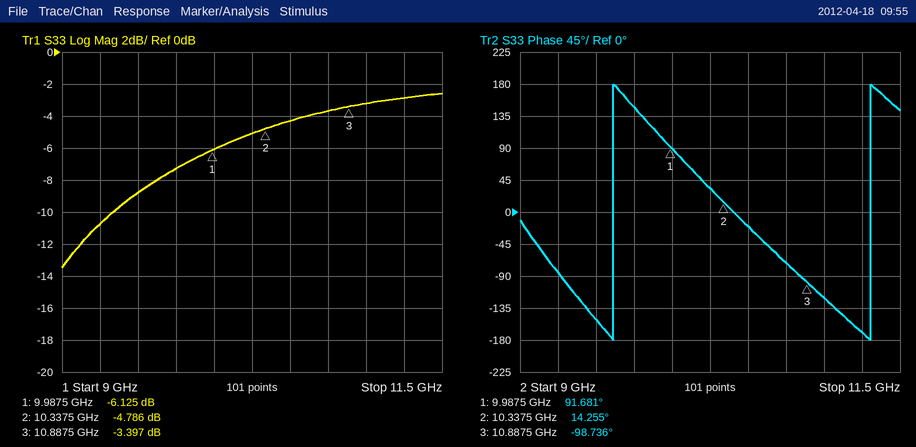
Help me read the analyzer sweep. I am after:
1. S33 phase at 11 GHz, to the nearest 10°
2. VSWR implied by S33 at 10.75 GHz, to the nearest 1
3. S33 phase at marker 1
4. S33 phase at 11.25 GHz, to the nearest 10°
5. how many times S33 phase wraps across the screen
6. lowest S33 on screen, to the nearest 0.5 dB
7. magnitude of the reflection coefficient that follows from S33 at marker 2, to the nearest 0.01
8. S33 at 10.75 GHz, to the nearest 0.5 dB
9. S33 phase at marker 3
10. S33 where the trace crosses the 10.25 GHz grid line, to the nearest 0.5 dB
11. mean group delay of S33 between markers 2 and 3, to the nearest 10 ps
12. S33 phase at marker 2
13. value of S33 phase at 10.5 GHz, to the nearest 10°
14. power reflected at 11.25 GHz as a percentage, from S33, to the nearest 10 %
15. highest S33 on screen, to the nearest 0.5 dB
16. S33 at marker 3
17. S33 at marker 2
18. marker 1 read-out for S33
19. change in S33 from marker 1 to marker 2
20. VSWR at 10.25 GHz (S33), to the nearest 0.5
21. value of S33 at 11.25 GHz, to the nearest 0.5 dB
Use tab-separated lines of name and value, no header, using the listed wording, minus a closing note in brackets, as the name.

S33 phase at 11 GHz, to the nearest 10°	-120°
VSWR implied by S33 at 10.75 GHz, to the nearest 1	5
S33 phase at marker 1	91.681°
S33 phase at 11.25 GHz, to the nearest 10°	-170°
how many times S33 phase wraps across the screen	2
lowest S33 on screen, to the nearest 0.5 dB	-13.5 dB
magnitude of the reflection coefficient that follows from S33 at marker 2, to the nearest 0.01	0.58
S33 at 10.75 GHz, to the nearest 0.5 dB	-3.5 dB
S33 phase at marker 3	-98.736°
S33 where the trace crosses the 10.25 GHz grid line, to the nearest 0.5 dB	-5.0 dB
mean group delay of S33 between markers 2 and 3, to the nearest 10 ps	570 ps
S33 phase at marker 2	14.255°
value of S33 phase at 10.5 GHz, to the nearest 10°	-20°
power reflected at 11.25 GHz as a percentage, from S33, to the nearest 10 %	50 %
highest S33 on screen, to the nearest 0.5 dB	-2.5 dB
S33 at marker 3	-3.397 dB
S33 at marker 2	-4.786 dB
marker 1 read-out for S33	-6.125 dB
change in S33 from marker 1 to marker 2	1.339 dB
VSWR at 10.25 GHz (S33), to the nearest 0.5	3.5
value of S33 at 11.25 GHz, to the nearest 0.5 dB	-3.0 dB
